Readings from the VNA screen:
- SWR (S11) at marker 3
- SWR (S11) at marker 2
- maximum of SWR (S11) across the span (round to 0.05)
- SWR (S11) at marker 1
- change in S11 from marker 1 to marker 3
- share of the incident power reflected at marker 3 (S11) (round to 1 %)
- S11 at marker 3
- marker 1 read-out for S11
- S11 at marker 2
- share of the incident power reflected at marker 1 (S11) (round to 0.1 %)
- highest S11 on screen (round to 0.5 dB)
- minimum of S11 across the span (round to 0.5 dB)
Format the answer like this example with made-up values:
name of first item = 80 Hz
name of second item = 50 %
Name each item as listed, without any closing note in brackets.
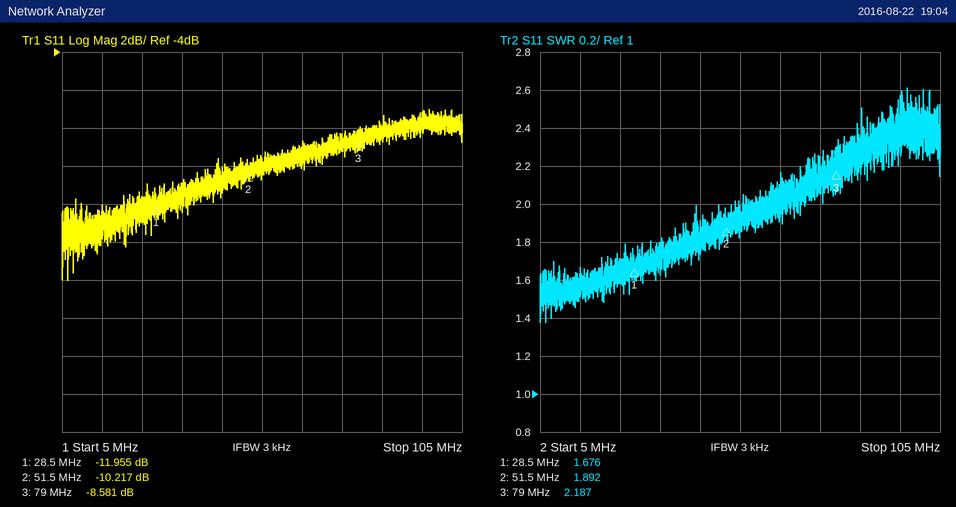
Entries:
SWR (S11) at marker 3 = 2.187
SWR (S11) at marker 2 = 1.892
maximum of SWR (S11) across the span = 2.60
SWR (S11) at marker 1 = 1.676
change in S11 from marker 1 to marker 3 = 3.374 dB
share of the incident power reflected at marker 3 (S11) = 14 %
S11 at marker 3 = -8.581 dB
marker 1 read-out for S11 = -11.955 dB
S11 at marker 2 = -10.217 dB
share of the incident power reflected at marker 1 (S11) = 6.4 %
highest S11 on screen = -7.0 dB
minimum of S11 across the span = -16.0 dB
